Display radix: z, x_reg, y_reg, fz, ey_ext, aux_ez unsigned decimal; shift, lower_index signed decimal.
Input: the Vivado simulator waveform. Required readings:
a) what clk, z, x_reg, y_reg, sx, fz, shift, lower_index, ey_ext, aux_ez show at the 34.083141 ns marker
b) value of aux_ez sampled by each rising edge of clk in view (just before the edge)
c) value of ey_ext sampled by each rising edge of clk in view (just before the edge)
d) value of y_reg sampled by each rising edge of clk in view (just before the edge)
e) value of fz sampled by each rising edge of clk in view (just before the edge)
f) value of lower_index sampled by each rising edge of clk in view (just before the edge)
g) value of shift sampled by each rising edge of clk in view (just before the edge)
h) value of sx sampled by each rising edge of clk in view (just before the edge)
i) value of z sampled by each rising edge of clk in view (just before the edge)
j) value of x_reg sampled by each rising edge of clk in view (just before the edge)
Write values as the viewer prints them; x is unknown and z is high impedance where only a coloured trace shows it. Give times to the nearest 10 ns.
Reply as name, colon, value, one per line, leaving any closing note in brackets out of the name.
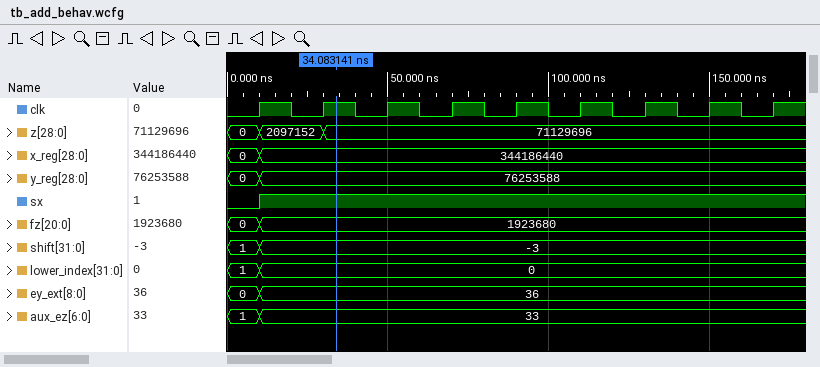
what clk, z, x_reg, y_reg, sx, fz, shift, lower_index, ey_ext, aux_ez show at the 34.083141 ns marker: clk=1, z=71129696, x_reg=344186440, y_reg=76253588, sx=1, fz=1923680, shift=-3, lower_index=0, ey_ext=36, aux_ez=33
value of aux_ez sampled by each rising edge of clk in view: 1, 33, 33, 33, 33, 33, 33, 33, 33
value of ey_ext sampled by each rising edge of clk in view: 0, 36, 36, 36, 36, 36, 36, 36, 36
value of y_reg sampled by each rising edge of clk in view: 0, 76253588, 76253588, 76253588, 76253588, 76253588, 76253588, 76253588, 76253588
value of fz sampled by each rising edge of clk in view: 0, 1923680, 1923680, 1923680, 1923680, 1923680, 1923680, 1923680, 1923680
value of lower_index sampled by each rising edge of clk in view: 1, 0, 0, 0, 0, 0, 0, 0, 0
value of shift sampled by each rising edge of clk in view: 1, -3, -3, -3, -3, -3, -3, -3, -3
value of sx sampled by each rising edge of clk in view: 0 1 1 1 1 1 1 1 1
value of z sampled by each rising edge of clk in view: 0, 2097152, 71129696, 71129696, 71129696, 71129696, 71129696, 71129696, 71129696
value of x_reg sampled by each rising edge of clk in view: 0, 344186440, 344186440, 344186440, 344186440, 344186440, 344186440, 344186440, 344186440
